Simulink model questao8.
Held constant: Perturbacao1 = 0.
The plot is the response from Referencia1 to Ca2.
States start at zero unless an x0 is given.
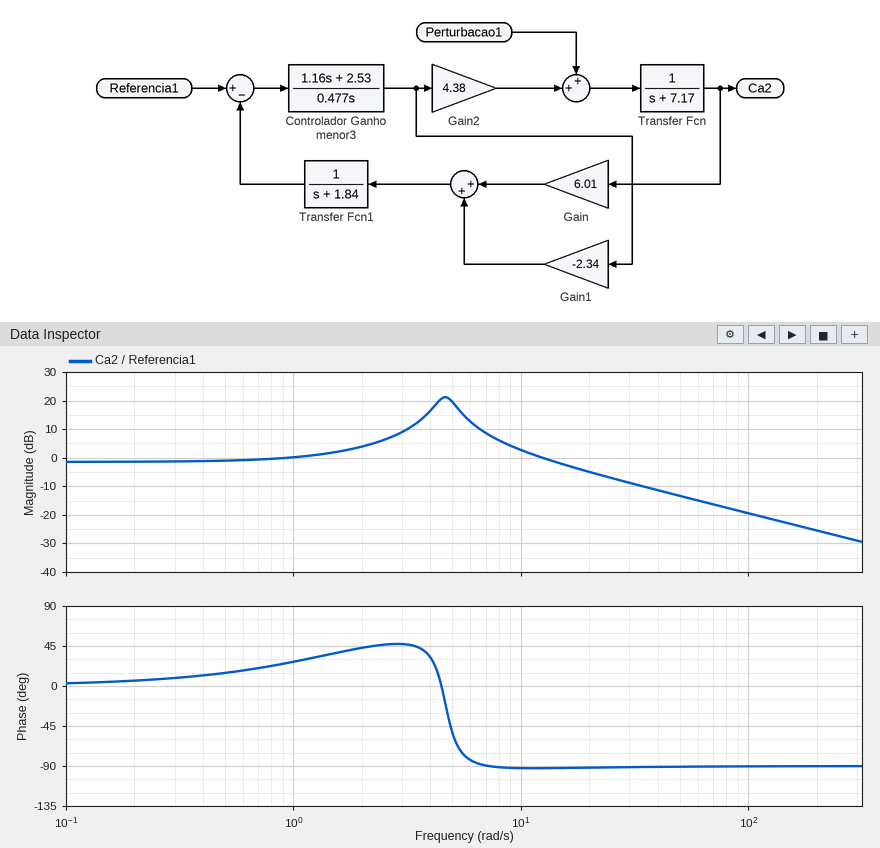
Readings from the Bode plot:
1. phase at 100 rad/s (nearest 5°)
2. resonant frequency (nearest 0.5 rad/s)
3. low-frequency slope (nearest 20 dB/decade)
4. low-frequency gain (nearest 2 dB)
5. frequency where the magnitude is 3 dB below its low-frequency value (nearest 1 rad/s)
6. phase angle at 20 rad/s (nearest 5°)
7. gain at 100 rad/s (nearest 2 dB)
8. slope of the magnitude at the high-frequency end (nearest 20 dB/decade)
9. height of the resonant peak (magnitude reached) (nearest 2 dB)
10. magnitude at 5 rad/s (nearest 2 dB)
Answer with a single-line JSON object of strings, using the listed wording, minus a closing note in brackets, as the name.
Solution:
{"phase at 100 rad/s": "-90°", "resonant frequency": "4.5 rad/s", "low-frequency slope": "0 dB/decade", "low-frequency gain": "-2 dB", "frequency where the magnitude is 3 dB below its low-frequency value": "19 rad/s", "phase angle at 20 rad/s": "-90°", "gain at 100 rad/s": "-20 dB", "slope of the magnitude at the high-frequency end": "-20 dB/decade", "height of the resonant peak (magnitude reached)": "22 dB", "magnitude at 5 rad/s": "20 dB"}
